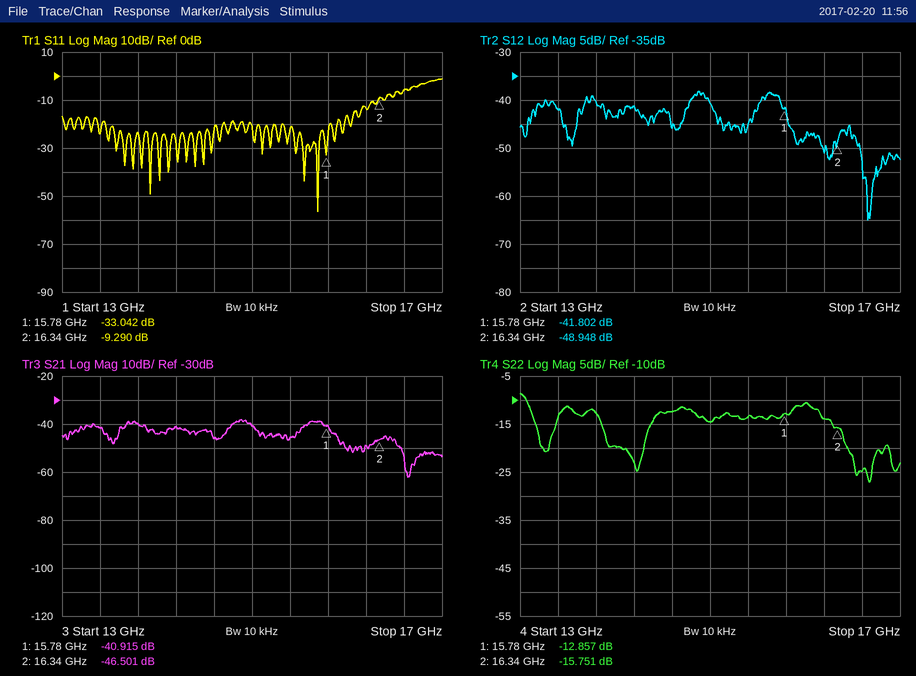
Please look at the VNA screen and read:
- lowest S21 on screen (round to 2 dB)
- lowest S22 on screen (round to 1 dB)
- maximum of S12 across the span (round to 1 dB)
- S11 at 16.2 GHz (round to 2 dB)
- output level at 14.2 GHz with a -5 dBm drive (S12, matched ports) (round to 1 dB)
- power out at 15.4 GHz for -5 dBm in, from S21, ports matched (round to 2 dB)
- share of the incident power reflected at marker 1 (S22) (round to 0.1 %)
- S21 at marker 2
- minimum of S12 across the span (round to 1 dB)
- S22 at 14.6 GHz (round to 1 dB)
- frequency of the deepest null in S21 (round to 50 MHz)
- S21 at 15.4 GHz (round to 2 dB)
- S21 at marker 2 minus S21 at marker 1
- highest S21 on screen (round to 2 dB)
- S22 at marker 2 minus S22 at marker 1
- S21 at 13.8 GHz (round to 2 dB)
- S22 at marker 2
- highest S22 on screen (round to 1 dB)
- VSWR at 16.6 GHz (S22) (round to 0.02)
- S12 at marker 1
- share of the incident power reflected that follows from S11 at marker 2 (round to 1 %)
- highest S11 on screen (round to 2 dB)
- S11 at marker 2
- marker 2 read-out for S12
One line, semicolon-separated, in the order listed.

-62 dB; -27 dB; -38 dB; -14 dB; -46 dBm; -50 dBm; 5.2 %; -46.501 dB; -65 dB; -12 dB; 16.65 GHz; -46 dB; -5.586 dB; -38 dB; -2.894 dB; -40 dB; -15.751 dB; -9 dB; 1.12; -41.802 dB; 12 %; -2 dB; -9.290 dB; -48.948 dB
